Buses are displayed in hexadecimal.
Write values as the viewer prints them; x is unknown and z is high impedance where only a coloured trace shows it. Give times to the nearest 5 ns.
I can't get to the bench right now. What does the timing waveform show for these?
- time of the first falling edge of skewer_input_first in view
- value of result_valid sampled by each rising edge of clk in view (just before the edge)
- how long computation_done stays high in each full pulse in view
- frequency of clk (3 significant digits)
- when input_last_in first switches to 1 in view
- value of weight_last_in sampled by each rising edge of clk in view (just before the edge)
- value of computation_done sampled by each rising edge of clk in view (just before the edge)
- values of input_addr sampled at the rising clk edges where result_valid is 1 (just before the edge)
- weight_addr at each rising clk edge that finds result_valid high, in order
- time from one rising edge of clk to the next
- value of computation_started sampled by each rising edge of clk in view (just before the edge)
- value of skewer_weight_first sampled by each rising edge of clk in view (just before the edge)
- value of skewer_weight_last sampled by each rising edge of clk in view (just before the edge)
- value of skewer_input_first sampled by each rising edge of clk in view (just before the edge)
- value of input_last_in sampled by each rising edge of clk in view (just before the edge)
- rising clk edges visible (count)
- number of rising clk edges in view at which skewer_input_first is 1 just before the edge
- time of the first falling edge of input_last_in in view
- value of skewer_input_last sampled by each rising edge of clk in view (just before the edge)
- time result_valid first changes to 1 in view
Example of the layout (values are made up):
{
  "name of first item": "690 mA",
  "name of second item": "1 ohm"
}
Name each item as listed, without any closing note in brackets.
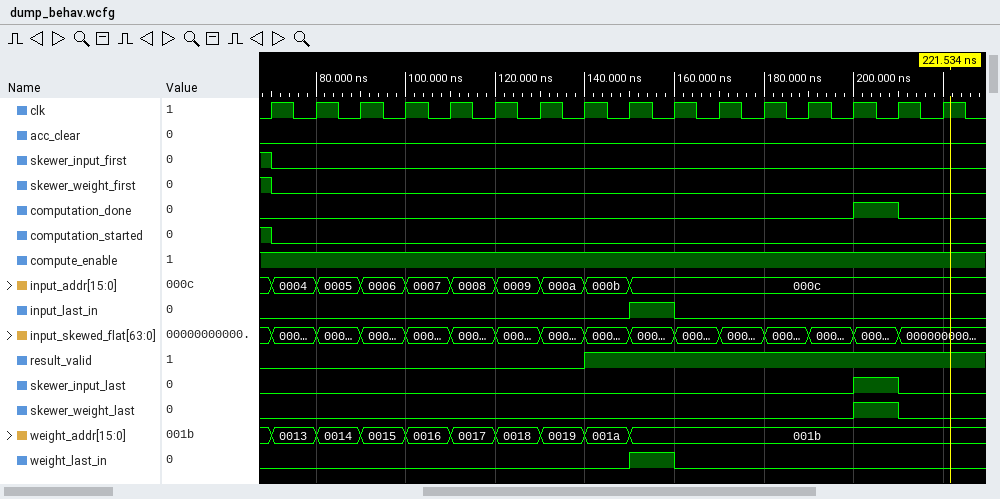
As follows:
{
  "time of the first falling edge of skewer_input_first in view": "70 ns",
  "value of result_valid sampled by each rising edge of clk in view": "0 0 0 0 0 0 0 0 1 1 1 1 1 1 1 1",
  "how long computation_done stays high in each full pulse in view": "10 ns",
  "frequency of clk": "100 MHz",
  "when input_last_in first switches to 1 in view": "150 ns",
  "value of weight_last_in sampled by each rising edge of clk in view": "0 0 0 0 0 0 0 0 0 1 0 0 0 0 0 0",
  "value of computation_done sampled by each rising edge of clk in view": "0 0 0 0 0 0 0 0 0 0 0 0 0 0 1 0",
  "values of input_addr sampled at the rising clk edges where result_valid is 1": "000b, 000c, 000c, 000c, 000c, 000c, 000c, 000c",
  "weight_addr at each rising clk edge that finds result_valid high, in order": "001a, 001b, 001b, 001b, 001b, 001b, 001b, 001b",
  "time from one rising edge of clk to the next": "10 ns",
  "value of computation_started sampled by each rising edge of clk in view": "1 0 0 0 0 0 0 0 0 0 0 0 0 0 0 0",
  "value of skewer_weight_first sampled by each rising edge of clk in view": "1 0 0 0 0 0 0 0 0 0 0 0 0 0 0 0",
  "value of skewer_weight_last sampled by each rising edge of clk in view": "0 0 0 0 0 0 0 0 0 0 0 0 0 0 1 0",
  "value of skewer_input_first sampled by each rising edge of clk in view": "1 0 0 0 0 0 0 0 0 0 0 0 0 0 0 0",
  "value of input_last_in sampled by each rising edge of clk in view": "0 0 0 0 0 0 0 0 0 1 0 0 0 0 0 0",
  "rising clk edges visible": "16",
  "number of rising clk edges in view at which skewer_input_first is 1 just before the edge": "1",
  "time of the first falling edge of input_last_in in view": "160 ns",
  "value of skewer_input_last sampled by each rising edge of clk in view": "0 0 0 0 0 0 0 0 0 0 0 0 0 0 1 0",
  "time result_valid first changes to 1 in view": "140 ns"
}
